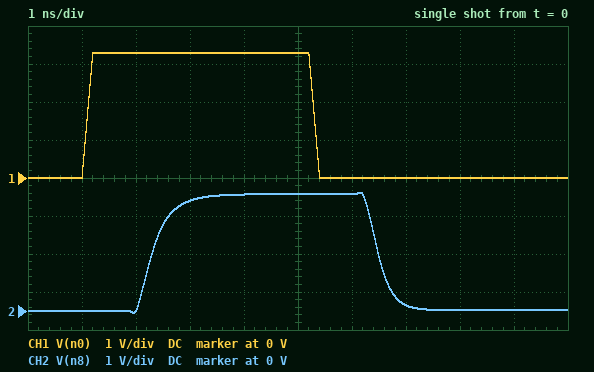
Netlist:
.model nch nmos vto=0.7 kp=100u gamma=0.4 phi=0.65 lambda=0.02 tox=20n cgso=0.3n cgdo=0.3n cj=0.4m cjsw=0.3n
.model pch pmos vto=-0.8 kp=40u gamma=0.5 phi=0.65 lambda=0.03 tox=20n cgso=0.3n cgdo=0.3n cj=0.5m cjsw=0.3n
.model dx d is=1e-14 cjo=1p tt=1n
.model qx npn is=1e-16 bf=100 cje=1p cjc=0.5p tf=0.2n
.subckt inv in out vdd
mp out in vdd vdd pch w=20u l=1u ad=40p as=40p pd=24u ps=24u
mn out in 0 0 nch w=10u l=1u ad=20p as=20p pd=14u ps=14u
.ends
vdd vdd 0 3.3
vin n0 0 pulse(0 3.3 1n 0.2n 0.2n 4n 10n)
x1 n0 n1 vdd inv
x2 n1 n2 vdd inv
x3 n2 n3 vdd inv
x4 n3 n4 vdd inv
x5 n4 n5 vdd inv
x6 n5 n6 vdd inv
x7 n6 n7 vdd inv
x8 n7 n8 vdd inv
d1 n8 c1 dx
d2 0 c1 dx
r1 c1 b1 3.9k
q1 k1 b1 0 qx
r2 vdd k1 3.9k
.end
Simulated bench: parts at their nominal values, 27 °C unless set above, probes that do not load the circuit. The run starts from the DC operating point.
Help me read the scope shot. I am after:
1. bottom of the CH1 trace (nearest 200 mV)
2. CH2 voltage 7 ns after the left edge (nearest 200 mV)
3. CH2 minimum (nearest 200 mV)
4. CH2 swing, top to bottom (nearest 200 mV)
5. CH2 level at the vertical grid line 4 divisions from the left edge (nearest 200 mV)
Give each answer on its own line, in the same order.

0 V
200 mV
0 V
3.2 V
3.0 V
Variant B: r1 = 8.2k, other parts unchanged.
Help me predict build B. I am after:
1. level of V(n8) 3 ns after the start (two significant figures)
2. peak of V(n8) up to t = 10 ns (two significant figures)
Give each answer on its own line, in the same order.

3.0 V
3.2 V
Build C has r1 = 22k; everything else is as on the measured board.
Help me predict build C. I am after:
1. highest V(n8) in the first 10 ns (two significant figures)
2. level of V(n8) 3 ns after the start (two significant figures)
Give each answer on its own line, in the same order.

3.3 V
3.1 V
